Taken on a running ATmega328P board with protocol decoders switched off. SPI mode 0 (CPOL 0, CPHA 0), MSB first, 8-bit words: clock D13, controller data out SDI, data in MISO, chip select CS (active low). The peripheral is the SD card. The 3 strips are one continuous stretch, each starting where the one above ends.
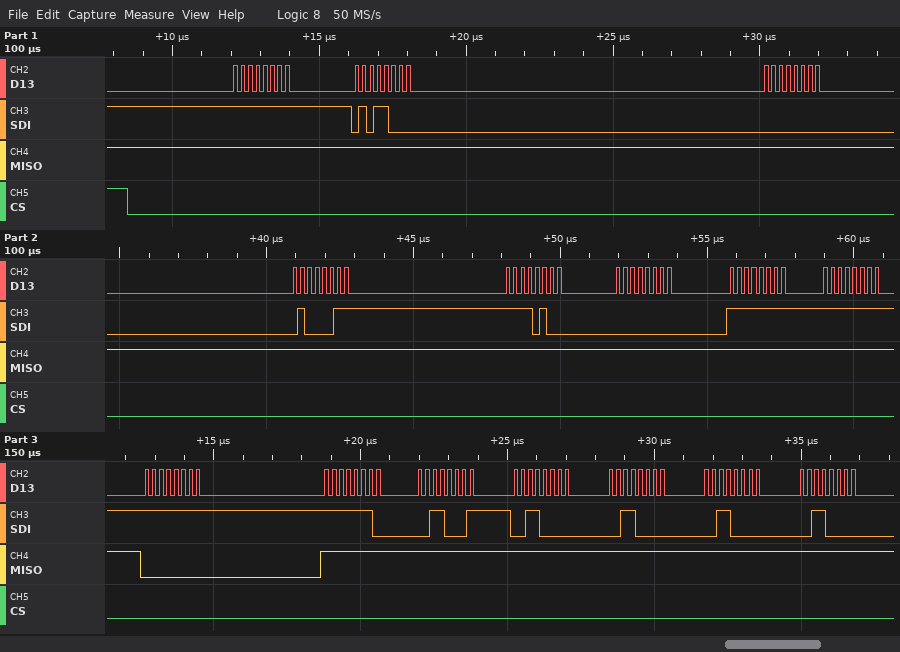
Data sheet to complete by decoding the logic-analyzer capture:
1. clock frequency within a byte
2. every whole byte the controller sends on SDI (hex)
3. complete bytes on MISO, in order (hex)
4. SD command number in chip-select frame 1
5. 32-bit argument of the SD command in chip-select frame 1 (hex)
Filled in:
4 MHz
FF 58 00 43 F4 00 FF FF FF FE 31 30 30 30 30
FF FF FF FF FF FF FF FF 00 FF FF FF FF FF FF
CMD24
0x0043F400
